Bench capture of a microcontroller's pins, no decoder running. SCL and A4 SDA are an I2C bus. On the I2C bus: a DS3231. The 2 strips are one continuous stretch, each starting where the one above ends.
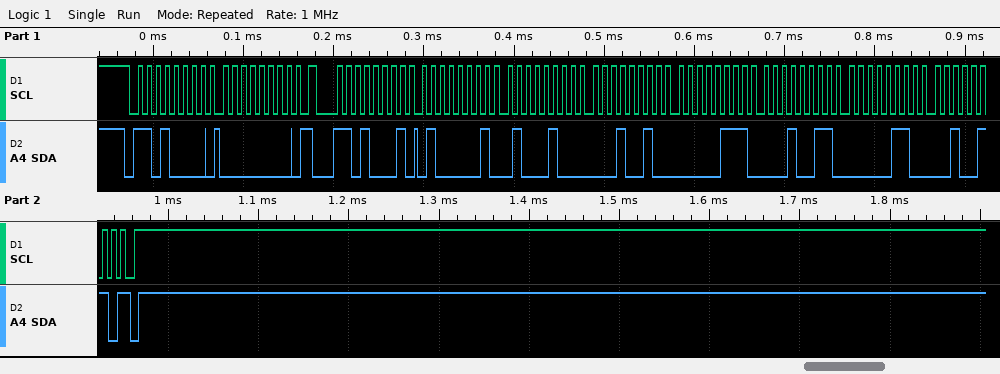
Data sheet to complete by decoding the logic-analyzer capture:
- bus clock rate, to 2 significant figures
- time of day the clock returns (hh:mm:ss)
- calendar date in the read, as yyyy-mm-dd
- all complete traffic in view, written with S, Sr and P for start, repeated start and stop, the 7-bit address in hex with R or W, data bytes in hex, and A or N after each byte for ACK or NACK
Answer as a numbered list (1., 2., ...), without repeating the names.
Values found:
1. 100 kHz
2. 12:44:41
3. 2026-06-13
4. S 68W A 00 A Sr 68R A 41 A 44 A 12 A 07 A 13 A 06 A 26 N P
